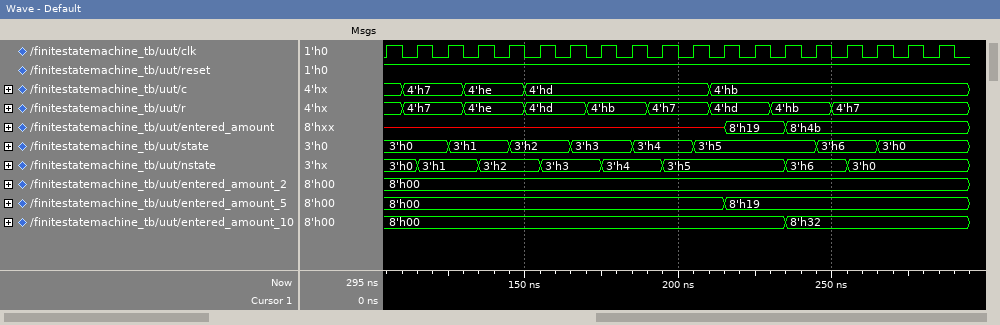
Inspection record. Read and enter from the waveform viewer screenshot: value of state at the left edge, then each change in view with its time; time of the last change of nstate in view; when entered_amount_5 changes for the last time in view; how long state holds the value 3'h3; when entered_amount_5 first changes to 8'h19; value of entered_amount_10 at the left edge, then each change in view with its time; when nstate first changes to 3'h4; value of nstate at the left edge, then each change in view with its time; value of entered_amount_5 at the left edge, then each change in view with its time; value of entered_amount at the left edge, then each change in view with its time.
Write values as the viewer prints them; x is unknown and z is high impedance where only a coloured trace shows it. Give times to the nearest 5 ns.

3'h0, 3'h1 at 125 ns, 3'h2 at 145 ns, 3'h3 at 165 ns, 3'h4 at 185 ns, 3'h5 at 205 ns, 3'h6 at 245 ns, 3'h0 at 265 ns
255 ns
215 ns
20 ns
215 ns
8'h00, 8'h32 at 235 ns
175 ns
3'h0, 3'h1 at 115 ns, 3'h2 at 135 ns, 3'h3 at 155 ns, 3'h4 at 175 ns, 3'h5 at 195 ns, 3'h6 at 235 ns, 3'h0 at 255 ns
8'h00, 8'h19 at 215 ns
x, 8'h19 at 215 ns, 8'h4b at 235 ns
